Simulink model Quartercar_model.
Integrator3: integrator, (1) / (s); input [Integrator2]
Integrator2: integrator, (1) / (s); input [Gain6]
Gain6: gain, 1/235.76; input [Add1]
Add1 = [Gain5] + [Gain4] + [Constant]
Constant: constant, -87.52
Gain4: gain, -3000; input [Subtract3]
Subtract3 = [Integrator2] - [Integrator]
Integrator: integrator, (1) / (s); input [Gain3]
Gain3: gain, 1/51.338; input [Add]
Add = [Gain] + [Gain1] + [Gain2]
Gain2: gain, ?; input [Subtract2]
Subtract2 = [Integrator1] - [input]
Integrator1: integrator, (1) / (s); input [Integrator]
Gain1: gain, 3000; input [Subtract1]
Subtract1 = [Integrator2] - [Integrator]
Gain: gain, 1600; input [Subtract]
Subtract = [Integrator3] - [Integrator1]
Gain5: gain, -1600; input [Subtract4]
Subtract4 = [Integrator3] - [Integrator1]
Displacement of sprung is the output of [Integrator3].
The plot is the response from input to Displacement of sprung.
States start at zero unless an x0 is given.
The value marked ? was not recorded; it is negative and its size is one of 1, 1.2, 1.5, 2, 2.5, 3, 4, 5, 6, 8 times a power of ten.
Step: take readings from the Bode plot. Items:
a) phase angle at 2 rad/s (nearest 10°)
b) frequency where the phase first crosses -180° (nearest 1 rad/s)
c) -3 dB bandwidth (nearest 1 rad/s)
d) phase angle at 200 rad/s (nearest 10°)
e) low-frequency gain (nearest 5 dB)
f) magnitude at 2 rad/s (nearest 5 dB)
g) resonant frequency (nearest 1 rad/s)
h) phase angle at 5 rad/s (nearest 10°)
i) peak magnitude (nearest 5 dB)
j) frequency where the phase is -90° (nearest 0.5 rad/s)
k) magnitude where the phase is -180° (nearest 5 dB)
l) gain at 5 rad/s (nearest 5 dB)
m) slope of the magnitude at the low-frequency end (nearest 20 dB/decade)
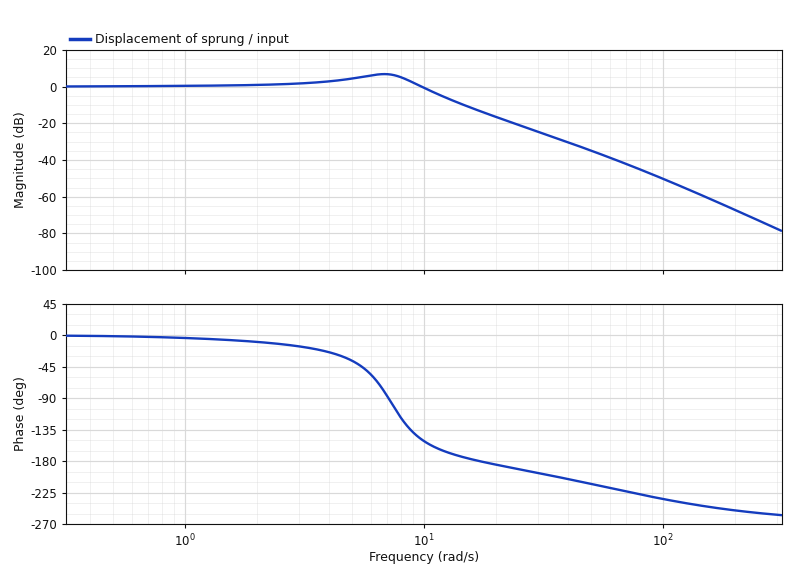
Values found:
-10°
17 rad/s
11 rad/s
-250°
0 dB
0 dB
7 rad/s
-40°
5 dB
7.0 rad/s
-15 dB
5 dB
0 dB/decade
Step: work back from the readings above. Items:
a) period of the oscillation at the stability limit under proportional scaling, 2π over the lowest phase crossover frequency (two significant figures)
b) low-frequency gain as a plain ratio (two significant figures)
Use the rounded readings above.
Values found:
0.37 s
1.0
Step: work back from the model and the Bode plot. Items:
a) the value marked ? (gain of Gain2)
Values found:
-15000
